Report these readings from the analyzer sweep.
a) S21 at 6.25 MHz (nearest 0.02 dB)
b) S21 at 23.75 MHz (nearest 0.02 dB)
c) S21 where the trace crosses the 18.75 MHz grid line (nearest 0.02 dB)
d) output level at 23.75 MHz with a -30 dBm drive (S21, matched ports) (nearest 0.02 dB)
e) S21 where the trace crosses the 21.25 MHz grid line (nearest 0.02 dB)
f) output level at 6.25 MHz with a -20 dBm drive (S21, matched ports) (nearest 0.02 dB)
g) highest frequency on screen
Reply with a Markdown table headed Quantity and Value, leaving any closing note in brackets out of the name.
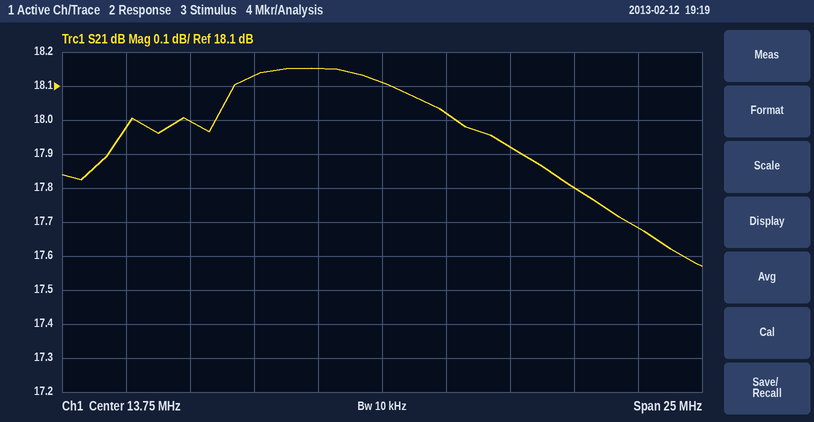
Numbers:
| Quantity | Value |
|---|---|
| S21 at 6.25 MHz | 18.00 dB |
| S21 at 23.75 MHz | 17.68 dB |
| S21 where the trace crosses the 18.75 MHz grid line | 17.92 dB |
| output level at 23.75 MHz with a -30 dBm drive (S21, matched ports) | -12.32 dBm |
| S21 where the trace crosses the 21.25 MHz grid line | 17.80 dB |
| output level at 6.25 MHz with a -20 dBm drive (S21, matched ports) | -2.00 dBm |
| highest frequency on screen | 26.25 MHz |
